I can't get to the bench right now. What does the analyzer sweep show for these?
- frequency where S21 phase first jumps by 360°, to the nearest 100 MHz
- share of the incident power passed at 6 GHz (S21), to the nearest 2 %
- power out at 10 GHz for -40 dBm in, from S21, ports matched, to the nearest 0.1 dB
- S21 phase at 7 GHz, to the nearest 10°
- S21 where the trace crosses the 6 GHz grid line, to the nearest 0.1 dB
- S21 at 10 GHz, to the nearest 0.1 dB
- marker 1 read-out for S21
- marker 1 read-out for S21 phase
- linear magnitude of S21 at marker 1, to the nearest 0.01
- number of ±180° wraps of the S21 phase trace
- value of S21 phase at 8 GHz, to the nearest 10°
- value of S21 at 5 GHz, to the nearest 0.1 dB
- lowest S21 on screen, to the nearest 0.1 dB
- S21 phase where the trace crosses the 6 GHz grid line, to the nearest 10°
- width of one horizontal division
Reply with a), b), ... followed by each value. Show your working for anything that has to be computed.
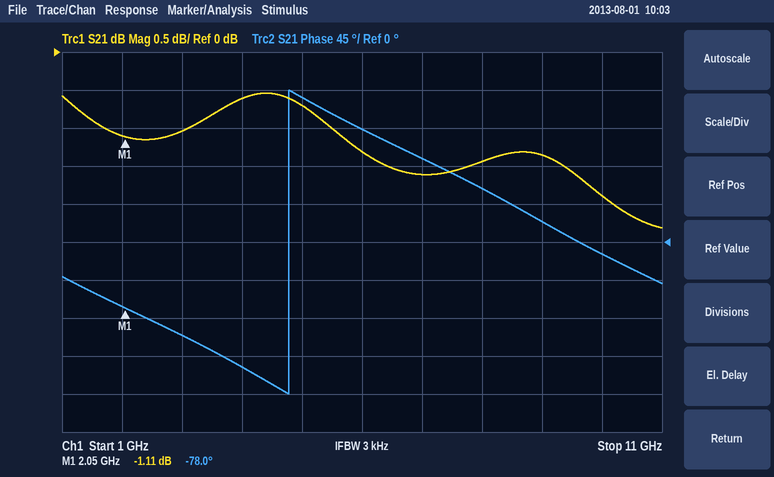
a) 4.8 GHz
b) 10^(-1.3/10) ≈ 74 %
c) -40 dBm + (-1.9 dB) = -41.9 dBm
d) 100°
e) -1.3 dB
f) -1.9 dB
g) -1.11 dB
h) -78.0°
i) 10^(-1.11/20) ≈ 0.88
j) 1
k) 60°
l) -0.7 dB
m) -2.3 dB
n) 130°
o) 1 GHz
